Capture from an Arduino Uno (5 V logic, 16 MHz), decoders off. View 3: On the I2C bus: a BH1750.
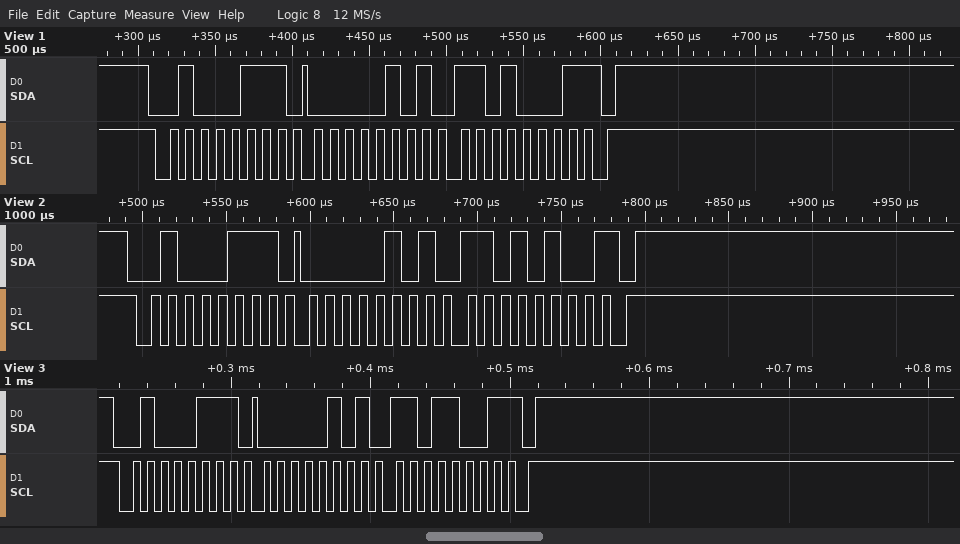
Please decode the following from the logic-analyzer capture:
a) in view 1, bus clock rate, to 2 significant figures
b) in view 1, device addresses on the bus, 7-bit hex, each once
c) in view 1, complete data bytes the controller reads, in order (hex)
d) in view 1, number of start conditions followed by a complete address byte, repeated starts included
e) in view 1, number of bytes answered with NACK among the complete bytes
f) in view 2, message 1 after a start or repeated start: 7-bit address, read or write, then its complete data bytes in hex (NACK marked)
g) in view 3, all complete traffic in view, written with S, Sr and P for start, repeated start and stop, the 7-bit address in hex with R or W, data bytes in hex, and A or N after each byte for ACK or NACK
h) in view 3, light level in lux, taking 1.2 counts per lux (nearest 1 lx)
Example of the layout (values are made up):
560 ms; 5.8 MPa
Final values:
100 kHz; 0x23; 05 D1; 1; 1; 0x23 read: 05 D4 NACK; S 23R A 05 A D9 N P; 1248 lx
